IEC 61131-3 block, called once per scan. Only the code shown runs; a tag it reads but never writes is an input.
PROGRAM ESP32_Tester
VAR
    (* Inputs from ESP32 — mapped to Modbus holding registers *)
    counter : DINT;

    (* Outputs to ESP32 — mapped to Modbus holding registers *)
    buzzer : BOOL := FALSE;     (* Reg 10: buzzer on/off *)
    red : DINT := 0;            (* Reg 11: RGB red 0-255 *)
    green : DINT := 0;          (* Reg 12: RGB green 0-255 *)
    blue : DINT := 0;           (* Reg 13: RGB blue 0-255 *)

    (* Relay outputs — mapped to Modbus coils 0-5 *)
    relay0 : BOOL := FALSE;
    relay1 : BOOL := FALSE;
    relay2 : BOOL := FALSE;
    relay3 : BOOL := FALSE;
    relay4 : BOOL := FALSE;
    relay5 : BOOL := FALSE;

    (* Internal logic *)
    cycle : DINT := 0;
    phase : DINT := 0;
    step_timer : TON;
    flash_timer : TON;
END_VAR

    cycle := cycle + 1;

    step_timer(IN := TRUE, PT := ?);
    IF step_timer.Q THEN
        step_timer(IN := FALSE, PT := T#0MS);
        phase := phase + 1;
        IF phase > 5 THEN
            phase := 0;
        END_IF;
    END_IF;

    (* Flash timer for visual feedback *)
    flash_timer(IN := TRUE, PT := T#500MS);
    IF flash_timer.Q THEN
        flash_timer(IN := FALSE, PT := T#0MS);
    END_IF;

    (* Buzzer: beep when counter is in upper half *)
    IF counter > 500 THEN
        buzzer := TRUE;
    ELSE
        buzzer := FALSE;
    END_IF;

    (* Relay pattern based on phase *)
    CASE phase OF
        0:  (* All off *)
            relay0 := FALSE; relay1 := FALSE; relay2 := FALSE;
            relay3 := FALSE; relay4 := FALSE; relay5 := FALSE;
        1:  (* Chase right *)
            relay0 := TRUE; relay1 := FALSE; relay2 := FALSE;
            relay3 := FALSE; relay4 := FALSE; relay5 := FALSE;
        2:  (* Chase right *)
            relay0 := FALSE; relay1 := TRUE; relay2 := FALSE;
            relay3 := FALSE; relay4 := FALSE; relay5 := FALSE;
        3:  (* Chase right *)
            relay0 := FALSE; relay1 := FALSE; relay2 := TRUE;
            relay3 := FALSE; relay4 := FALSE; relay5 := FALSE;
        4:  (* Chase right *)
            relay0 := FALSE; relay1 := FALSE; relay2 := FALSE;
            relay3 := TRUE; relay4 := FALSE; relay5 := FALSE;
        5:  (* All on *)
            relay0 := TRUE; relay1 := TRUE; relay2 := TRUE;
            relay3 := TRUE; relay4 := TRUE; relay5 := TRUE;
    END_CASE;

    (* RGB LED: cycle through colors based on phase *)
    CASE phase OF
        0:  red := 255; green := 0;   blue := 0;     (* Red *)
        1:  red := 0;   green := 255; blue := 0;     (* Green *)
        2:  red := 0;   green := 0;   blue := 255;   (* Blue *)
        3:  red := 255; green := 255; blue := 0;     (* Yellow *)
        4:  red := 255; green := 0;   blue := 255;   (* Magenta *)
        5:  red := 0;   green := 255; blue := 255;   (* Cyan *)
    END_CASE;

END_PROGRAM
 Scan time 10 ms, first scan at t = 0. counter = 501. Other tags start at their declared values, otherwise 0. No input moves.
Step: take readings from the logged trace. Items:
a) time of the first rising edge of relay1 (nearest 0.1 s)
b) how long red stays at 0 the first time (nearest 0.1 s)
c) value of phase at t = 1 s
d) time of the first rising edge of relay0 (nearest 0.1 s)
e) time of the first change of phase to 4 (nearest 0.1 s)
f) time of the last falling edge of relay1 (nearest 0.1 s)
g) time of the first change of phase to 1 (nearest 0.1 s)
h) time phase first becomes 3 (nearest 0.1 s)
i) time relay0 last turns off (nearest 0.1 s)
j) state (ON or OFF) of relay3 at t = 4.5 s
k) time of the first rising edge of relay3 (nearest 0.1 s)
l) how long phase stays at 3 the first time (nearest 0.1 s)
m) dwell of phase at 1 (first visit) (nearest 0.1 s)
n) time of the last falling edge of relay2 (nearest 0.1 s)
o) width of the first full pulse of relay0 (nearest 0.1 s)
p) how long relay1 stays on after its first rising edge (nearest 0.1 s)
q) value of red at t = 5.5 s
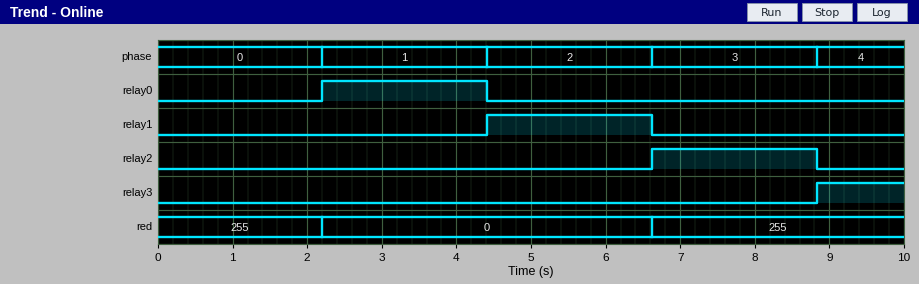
4.4 s
4.4 s
0
2.2 s
8.8 s
6.6 s
2.2 s
6.6 s
4.4 s
OFF
8.8 s
2.2 s
2.2 s
8.8 s
2.2 s
2.2 s
0
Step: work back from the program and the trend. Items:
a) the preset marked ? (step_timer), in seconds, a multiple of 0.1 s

2.2 s
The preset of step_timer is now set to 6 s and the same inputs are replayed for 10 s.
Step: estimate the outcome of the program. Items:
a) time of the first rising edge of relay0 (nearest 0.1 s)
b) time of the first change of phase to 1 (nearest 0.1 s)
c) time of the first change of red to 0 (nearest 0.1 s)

6.0 s
6.0 s
6.0 s
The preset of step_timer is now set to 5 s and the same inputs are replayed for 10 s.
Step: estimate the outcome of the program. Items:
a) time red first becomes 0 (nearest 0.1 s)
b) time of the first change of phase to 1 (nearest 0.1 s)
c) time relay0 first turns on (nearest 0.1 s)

5.0 s
5.0 s
5.0 s
